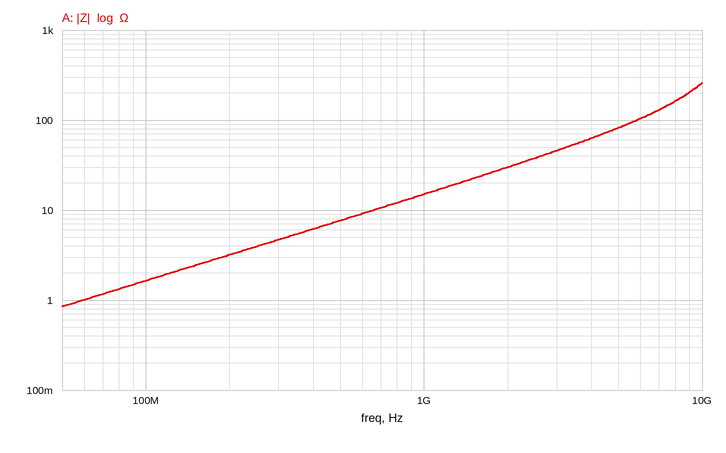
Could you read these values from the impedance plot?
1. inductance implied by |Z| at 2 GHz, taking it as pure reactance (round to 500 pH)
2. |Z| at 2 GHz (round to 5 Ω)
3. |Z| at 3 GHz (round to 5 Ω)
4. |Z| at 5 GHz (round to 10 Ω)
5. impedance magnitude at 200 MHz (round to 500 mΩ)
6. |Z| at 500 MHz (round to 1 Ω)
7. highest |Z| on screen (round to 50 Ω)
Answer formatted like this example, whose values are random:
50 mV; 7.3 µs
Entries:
2.5 nH; 30 Ω; 45 Ω; 80 Ω; 3.0 Ω; 8 Ω; 250 Ω
